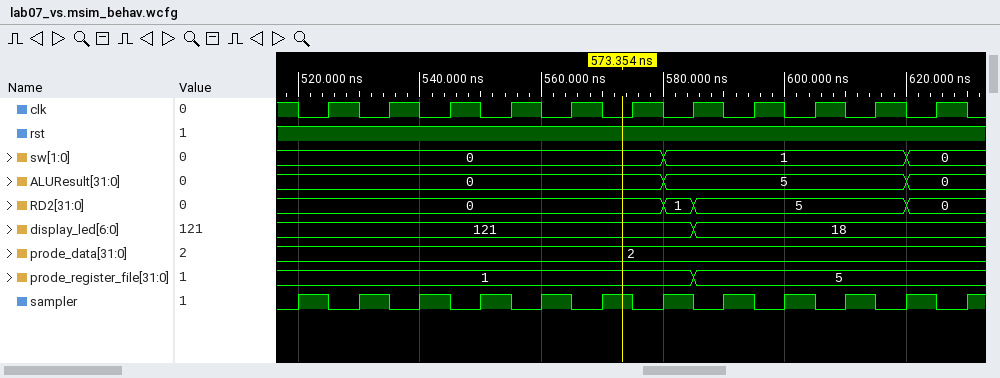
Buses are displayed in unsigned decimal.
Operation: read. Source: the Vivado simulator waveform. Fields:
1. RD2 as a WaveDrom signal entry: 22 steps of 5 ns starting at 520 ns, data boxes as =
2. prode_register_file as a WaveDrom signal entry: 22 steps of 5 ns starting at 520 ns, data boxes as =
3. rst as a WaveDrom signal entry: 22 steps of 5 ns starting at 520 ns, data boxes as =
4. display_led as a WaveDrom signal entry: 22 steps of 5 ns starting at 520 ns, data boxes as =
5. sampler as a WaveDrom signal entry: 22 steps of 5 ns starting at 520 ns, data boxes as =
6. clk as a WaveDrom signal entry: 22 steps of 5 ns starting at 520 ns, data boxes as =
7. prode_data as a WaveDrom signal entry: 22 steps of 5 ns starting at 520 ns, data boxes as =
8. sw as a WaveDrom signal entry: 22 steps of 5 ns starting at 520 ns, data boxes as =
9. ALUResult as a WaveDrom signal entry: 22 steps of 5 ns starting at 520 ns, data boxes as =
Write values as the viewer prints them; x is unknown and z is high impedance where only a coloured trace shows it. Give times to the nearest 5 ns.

{name: 'RD2', wave: '=...........==......=.', data: '0 1 5 0'}
{name: 'prode_register_file', wave: '=............=........', data: '1 5'}
{name: 'rst', wave: '1.....................'}
{name: 'display_led', wave: '=............=........', data: '121 18'}
{name: 'sampler', wave: '1010101010101010101010'}
{name: 'clk', wave: '0101010101010101010101'}
{name: 'prode_data', wave: '=.....................', data: '2'}
{name: 'sw', wave: '=...........=.......=.', data: '0 1 0'}
{name: 'ALUResult', wave: '=...........=.......=.', data: '0 5 0'}
